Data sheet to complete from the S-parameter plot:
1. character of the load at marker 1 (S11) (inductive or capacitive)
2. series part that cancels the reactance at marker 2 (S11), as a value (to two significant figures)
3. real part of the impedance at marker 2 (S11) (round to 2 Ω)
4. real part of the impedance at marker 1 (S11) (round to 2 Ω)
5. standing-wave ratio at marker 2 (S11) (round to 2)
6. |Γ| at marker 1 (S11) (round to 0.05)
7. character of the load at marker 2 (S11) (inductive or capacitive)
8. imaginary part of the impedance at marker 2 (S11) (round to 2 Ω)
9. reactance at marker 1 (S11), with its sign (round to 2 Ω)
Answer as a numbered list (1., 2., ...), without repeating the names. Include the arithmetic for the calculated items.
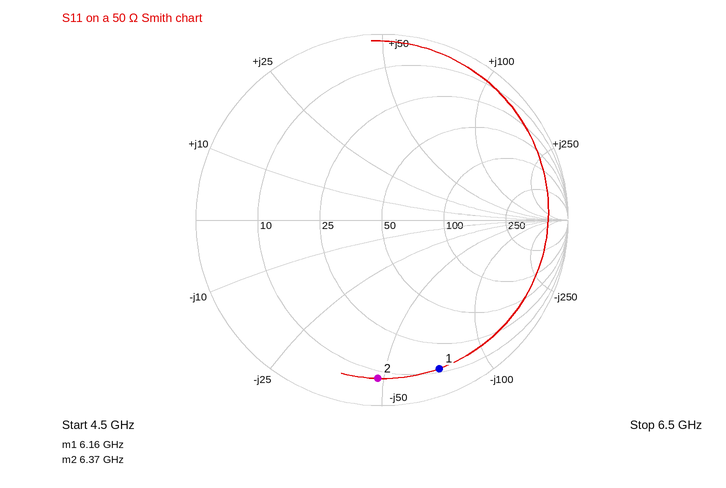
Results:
1. capacitive
2. L = 48 Ω/(2π × 6.37 GHz) ≈ 1.2 nH
3. 8 Ω
4. 12 Ω
5. 12
6. 0.85
7. capacitive
8. -48 Ω
9. -72 Ω
